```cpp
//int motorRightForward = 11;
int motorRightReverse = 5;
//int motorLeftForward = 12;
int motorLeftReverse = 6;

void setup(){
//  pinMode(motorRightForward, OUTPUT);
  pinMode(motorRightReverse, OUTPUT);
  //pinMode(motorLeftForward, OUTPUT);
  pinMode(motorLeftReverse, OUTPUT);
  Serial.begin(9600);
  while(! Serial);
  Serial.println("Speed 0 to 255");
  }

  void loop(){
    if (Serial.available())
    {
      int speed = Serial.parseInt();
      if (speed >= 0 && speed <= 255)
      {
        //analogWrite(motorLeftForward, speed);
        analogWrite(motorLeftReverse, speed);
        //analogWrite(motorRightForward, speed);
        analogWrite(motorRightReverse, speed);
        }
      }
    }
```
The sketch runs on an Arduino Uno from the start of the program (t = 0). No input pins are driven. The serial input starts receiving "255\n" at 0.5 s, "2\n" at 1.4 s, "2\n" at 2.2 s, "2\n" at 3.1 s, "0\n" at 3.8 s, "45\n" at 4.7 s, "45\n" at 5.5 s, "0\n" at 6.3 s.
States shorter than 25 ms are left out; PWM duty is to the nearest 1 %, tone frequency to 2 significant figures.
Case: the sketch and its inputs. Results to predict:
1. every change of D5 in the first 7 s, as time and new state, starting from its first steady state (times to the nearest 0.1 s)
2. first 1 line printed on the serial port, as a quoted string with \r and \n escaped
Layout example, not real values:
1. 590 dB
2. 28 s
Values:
1. 0 s low; 0.5 s high; 1.4 s PWM 1 %; 3.8 s low; 4.7 s PWM 18 %; 6.3 s low
2. "Speed 0 to 255\r\n"
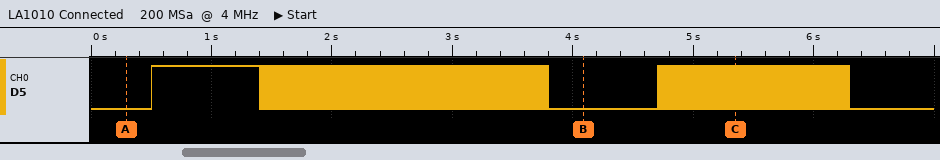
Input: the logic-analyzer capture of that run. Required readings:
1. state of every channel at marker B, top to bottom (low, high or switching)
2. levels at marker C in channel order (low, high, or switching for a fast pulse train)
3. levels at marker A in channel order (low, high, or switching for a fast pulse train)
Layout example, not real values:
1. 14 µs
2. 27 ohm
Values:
1. D5 low
2. D5 switching
3. D5 low
